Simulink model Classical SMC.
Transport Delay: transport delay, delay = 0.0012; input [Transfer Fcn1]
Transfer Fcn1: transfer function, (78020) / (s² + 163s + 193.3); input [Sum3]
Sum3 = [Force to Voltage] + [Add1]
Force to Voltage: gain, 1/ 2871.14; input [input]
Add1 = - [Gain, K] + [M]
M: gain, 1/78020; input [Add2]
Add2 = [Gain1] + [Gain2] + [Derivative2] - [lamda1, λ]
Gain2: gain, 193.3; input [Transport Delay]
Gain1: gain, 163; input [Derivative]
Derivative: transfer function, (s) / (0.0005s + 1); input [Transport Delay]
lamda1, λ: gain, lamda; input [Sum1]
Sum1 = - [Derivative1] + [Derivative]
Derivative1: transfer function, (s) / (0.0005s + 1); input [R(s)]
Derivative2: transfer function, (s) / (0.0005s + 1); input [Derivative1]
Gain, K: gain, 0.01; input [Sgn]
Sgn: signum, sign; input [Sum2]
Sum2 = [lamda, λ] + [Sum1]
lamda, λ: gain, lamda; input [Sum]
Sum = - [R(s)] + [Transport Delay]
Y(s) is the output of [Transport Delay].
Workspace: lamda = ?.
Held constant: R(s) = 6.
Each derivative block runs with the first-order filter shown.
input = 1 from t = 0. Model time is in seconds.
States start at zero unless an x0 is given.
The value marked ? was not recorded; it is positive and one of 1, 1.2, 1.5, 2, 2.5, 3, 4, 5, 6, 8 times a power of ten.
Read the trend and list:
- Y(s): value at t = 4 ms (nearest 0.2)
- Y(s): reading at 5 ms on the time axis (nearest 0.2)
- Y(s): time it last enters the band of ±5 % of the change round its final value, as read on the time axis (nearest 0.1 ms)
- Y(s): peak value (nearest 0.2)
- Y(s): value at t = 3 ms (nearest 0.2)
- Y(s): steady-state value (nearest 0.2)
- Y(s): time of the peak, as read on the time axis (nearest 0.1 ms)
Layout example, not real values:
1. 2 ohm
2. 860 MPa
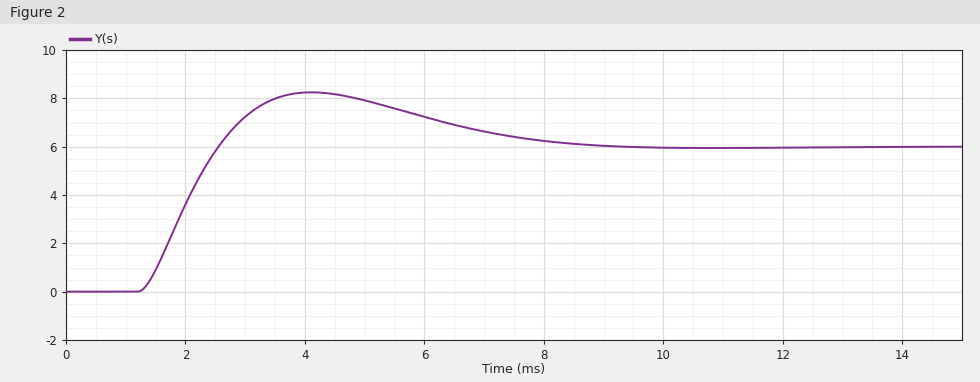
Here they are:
1. 8.2
2. 8.0
3. 7.8 ms
4. 8.2
5. 7.2
6. 6.0
7. 4.1 ms
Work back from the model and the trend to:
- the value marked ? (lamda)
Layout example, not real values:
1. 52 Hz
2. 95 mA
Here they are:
1. 400
